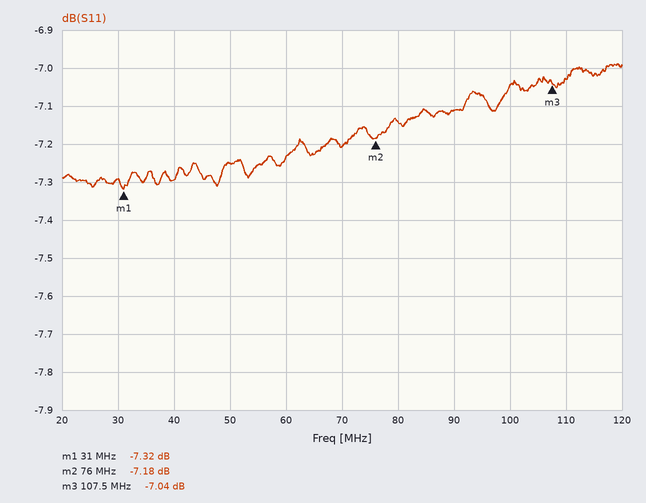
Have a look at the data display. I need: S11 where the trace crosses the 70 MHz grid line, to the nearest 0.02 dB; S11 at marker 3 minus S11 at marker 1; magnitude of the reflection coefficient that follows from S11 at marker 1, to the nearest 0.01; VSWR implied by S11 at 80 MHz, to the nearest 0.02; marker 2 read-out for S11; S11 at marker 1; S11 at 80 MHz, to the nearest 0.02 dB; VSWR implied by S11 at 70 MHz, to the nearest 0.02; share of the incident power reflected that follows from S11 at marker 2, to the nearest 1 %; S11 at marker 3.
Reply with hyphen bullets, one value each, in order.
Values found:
- -7.20 dB
- 0.28 dB
- 0.43
- 2.56
- -7.18 dB
- -7.32 dB
- -7.14 dB
- 2.54
- 19 %
- -7.04 dB
